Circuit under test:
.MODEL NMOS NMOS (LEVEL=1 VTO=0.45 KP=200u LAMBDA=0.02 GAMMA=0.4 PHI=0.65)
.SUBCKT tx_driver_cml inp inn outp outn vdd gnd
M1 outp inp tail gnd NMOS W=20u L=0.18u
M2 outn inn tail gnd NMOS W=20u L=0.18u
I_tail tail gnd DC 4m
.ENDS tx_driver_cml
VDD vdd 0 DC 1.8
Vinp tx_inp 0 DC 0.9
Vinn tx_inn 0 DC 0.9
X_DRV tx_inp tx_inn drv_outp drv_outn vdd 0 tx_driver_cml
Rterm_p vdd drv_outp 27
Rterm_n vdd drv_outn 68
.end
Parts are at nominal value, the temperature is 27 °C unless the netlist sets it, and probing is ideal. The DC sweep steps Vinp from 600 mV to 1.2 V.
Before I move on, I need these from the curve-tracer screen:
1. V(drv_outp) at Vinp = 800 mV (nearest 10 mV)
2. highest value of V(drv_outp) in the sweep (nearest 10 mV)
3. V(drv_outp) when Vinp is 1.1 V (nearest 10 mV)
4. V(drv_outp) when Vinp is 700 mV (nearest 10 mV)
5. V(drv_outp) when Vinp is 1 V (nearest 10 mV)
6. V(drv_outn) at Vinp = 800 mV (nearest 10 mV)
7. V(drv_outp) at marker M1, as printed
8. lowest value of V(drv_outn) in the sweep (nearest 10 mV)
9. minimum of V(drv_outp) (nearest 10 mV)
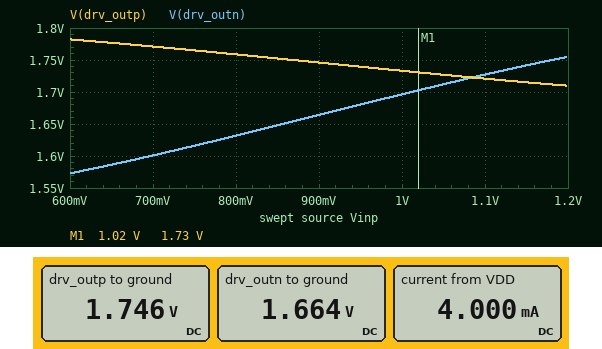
1.76 V
1.78 V
1.72 V
1.77 V
1.73 V
1.63 V
1.73 V
1.57 V
1.71 V
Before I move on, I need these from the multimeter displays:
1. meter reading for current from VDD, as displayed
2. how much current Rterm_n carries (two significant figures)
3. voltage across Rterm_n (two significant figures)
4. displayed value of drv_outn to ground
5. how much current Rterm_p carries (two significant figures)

4.000 mA
2.0 mA
140 mV
1.664 V
2.0 mA
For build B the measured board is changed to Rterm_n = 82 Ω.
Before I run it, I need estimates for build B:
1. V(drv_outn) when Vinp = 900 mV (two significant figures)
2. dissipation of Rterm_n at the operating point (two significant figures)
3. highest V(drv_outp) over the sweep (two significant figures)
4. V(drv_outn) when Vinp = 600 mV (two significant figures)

1.6 V
330 µW
1.8 V
1.5 V
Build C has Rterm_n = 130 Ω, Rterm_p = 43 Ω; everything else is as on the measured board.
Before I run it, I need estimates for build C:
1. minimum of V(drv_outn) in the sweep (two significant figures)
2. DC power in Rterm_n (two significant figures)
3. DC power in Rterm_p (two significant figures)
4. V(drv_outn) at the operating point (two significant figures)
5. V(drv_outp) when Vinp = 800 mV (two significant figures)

1.4 V
520 µW
170 µW
1.5 V
1.7 V
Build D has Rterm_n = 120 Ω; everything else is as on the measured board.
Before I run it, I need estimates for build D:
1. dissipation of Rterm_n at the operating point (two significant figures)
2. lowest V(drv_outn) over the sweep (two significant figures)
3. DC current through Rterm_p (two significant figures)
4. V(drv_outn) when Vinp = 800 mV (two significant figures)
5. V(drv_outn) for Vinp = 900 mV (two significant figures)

480 µW
1.4 V
2.0 mA
1.5 V
1.6 V
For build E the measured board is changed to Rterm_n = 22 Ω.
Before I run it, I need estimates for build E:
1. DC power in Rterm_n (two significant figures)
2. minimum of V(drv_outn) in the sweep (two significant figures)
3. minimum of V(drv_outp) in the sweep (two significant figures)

88 µW
1.7 V
1.7 V
